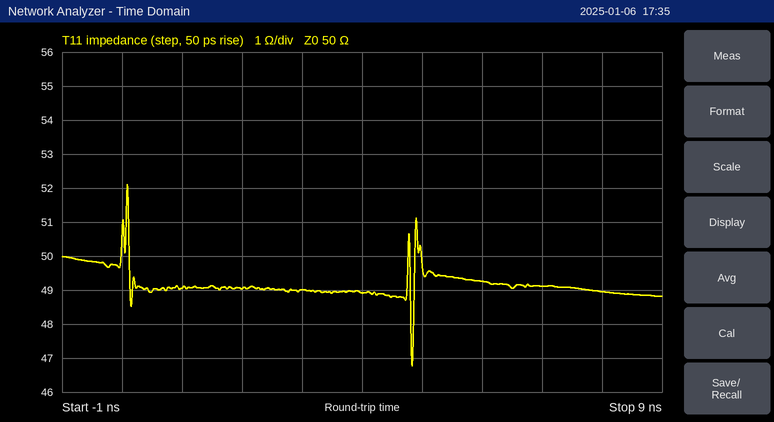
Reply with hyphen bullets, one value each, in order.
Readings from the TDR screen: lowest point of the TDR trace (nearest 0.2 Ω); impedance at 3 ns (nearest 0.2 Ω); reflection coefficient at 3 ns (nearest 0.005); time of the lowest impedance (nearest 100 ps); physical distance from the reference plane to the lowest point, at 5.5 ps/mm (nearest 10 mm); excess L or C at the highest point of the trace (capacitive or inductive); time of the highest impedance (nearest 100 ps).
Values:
- 46.8 Ω
- 49.0 Ω
- -0.010
- 4.8 ns
- 440 mm
- inductive
- 100 ps
